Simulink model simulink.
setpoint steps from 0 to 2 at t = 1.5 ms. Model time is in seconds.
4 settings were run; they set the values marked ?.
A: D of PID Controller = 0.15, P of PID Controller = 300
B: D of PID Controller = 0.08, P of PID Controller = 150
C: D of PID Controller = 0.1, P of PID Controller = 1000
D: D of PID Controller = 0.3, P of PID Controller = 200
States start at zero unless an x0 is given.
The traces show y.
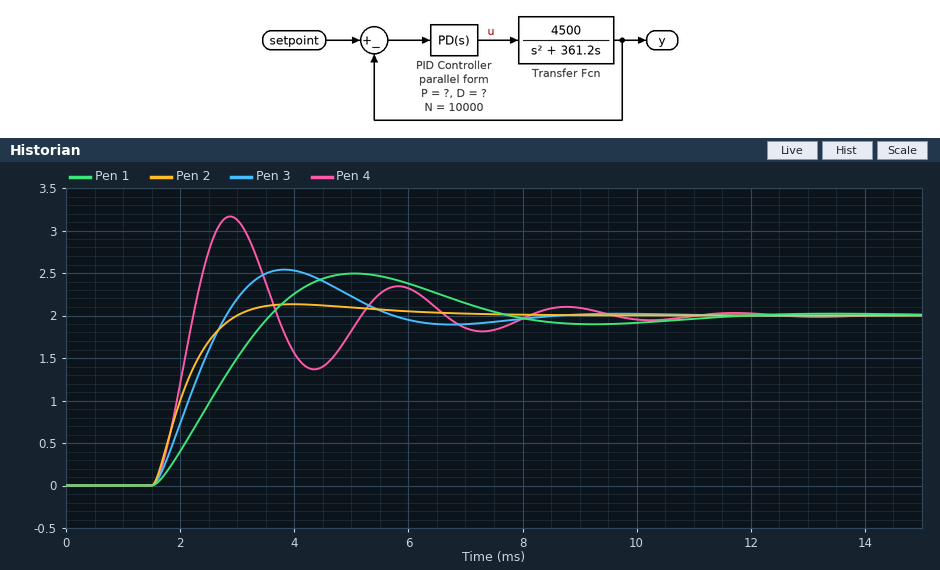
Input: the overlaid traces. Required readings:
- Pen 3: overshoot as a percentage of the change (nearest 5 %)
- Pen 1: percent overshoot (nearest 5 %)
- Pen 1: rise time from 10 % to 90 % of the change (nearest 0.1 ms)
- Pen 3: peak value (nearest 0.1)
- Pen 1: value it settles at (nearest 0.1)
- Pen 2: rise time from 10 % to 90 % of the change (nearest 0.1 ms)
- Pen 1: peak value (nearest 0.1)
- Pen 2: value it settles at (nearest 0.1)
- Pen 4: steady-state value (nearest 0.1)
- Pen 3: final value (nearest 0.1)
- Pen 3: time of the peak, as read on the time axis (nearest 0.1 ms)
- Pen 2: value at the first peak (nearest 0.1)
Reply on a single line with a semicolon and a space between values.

25 %; 25 %; 1.5 ms; 2.5; 2.0; 1.0 ms; 2.5; 2.0; 2.0; 2.0; 3.8 ms; 2.1
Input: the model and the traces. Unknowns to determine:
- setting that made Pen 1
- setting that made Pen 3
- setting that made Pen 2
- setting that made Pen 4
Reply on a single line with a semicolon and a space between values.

B; A; D; C
